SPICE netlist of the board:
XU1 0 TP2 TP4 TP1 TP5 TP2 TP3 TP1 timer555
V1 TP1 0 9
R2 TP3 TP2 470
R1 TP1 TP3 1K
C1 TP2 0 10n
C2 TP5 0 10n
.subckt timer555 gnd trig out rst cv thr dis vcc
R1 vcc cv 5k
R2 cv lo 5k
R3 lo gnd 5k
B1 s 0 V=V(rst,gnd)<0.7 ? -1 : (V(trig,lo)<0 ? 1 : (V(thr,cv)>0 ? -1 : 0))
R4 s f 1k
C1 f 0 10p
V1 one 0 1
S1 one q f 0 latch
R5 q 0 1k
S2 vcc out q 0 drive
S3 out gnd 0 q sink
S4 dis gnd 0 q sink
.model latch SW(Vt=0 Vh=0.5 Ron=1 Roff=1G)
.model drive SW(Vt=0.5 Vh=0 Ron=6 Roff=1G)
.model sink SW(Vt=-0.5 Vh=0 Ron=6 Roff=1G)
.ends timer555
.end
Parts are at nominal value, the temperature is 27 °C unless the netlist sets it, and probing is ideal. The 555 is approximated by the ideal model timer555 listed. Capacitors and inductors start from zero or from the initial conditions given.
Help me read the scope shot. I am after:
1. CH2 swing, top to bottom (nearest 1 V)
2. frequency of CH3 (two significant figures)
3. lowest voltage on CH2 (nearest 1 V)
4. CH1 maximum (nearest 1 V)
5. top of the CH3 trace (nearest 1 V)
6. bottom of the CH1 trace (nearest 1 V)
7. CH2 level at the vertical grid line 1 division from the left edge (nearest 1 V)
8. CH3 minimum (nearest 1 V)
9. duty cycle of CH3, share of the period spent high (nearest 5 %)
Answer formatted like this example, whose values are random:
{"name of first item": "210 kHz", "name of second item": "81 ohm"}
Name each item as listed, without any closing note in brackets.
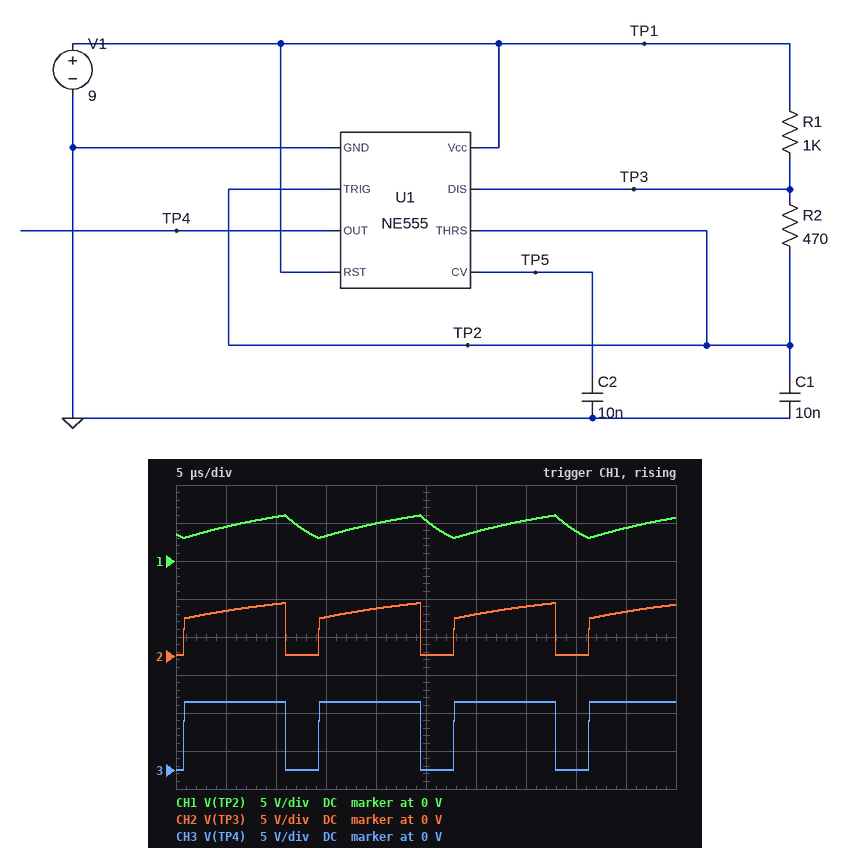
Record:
{"CH2 swing, top to bottom": "7 V", "frequency of CH3": "74 kHz", "lowest voltage on CH2": "0 V", "CH1 maximum": "6 V", "top of the CH3 trace": "9 V", "bottom of the CH1 trace": "3 V", "CH2 level at the vertical grid line 1 division from the left edge": "6 V", "CH3 minimum": "0 V", "duty cycle of CH3, share of the period spent high": "75 %"}
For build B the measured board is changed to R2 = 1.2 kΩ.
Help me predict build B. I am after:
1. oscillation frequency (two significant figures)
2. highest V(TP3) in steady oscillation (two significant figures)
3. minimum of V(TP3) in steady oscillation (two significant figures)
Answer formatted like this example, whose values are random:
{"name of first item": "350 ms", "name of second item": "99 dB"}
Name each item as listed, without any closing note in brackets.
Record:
{"oscillation frequency": "42 kHz", "highest V(TP3) in steady oscillation": "7.6 V", "minimum of V(TP3) in steady oscillation": "68 mV"}
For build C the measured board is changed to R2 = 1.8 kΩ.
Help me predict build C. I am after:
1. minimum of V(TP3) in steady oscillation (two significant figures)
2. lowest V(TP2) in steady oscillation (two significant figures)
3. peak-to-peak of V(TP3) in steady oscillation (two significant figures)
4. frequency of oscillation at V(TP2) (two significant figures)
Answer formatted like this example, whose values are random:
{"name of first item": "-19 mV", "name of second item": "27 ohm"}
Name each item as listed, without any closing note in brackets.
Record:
{"minimum of V(TP3) in steady oscillation": "63 mV", "lowest V(TP2) in steady oscillation": "3.0 V", "peak-to-peak of V(TP3) in steady oscillation": "7.9 V", "frequency of oscillation at V(TP2)": "31 kHz"}
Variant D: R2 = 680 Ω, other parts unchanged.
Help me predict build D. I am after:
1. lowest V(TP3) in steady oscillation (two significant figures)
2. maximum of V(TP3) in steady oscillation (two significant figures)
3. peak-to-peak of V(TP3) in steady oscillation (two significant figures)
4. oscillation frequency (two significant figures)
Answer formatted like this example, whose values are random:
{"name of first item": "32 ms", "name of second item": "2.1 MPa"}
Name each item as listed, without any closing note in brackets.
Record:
{"lowest V(TP3) in steady oscillation": "79 mV", "maximum of V(TP3) in steady oscillation": "7.2 V", "peak-to-peak of V(TP3) in steady oscillation": "7.1 V", "oscillation frequency": "61 kHz"}
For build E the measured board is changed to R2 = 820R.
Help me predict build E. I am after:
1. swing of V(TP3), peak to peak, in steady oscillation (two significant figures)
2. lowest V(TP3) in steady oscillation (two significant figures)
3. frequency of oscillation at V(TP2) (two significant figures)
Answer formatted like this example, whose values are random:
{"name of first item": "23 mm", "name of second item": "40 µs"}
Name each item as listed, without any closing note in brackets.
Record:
{"swing of V(TP3), peak to peak, in steady oscillation": "7.3 V", "lowest V(TP3) in steady oscillation": "75 mV", "frequency of oscillation at V(TP2)": "54 kHz"}
